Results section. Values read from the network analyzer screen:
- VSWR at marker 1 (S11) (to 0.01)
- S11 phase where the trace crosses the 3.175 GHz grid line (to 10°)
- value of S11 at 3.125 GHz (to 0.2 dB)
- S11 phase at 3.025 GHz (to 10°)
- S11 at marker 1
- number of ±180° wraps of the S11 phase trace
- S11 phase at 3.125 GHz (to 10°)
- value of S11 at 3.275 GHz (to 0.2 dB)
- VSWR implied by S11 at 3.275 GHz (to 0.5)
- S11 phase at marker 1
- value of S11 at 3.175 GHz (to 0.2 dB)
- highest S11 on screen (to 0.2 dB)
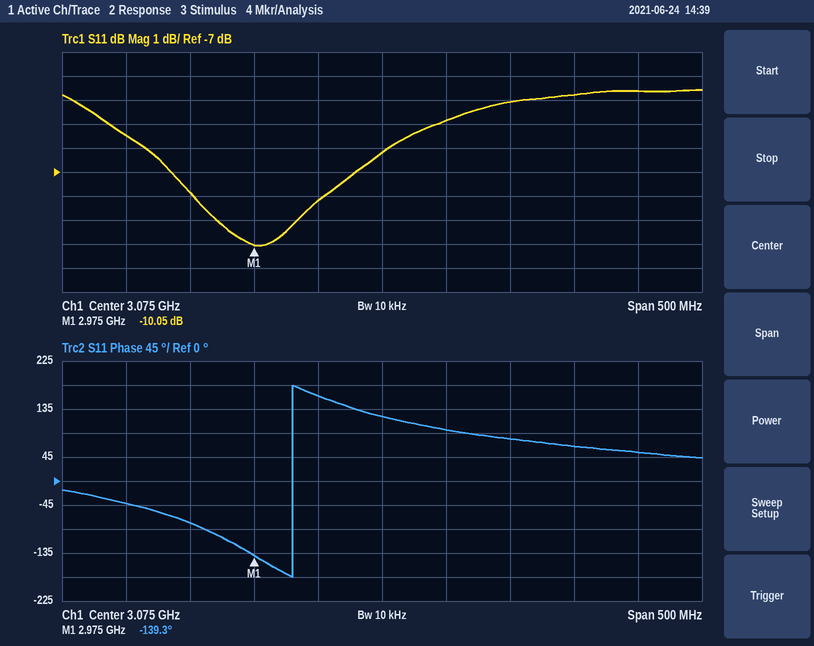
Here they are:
1.92
80°
-4.8 dB
160°
-10.05 dB
1
100°
-3.6 dB
5.0
-139.3°
-4.0 dB
-3.6 dB
